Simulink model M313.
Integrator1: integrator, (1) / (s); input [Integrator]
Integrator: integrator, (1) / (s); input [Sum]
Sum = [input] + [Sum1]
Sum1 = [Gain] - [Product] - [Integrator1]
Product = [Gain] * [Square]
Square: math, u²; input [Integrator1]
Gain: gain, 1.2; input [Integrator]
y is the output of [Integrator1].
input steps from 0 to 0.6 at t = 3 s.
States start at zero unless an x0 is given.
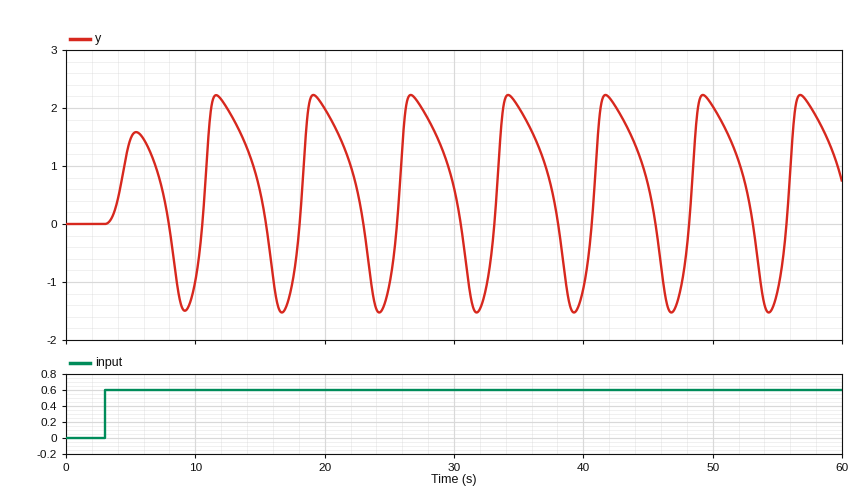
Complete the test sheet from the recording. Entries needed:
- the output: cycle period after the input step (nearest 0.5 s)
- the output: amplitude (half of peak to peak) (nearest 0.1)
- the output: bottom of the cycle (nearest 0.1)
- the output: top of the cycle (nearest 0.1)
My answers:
7.5 s
1.9
-1.5
2.2
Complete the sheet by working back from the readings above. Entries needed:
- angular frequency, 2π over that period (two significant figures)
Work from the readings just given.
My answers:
0.84 rad/s
